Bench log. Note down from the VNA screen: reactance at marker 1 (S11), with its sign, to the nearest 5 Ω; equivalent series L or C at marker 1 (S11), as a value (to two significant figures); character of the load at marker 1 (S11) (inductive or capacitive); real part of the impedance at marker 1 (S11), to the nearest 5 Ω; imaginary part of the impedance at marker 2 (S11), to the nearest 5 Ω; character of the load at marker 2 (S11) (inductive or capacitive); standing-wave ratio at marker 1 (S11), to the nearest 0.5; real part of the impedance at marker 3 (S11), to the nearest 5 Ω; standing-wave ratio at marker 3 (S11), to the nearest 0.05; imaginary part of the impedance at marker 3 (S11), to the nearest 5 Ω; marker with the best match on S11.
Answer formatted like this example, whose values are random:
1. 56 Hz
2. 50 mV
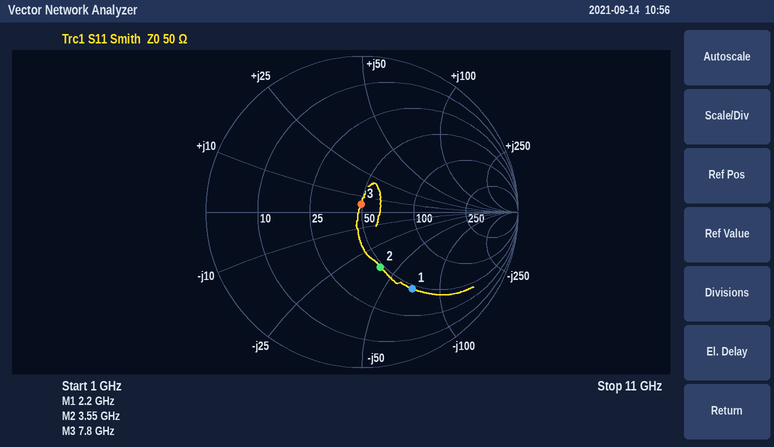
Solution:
1. -70 Ω
2. 1.0 pF
3. capacitive
4. 45 Ω
5. -40 Ω
6. capacitive
7. 4.0
8. 50 Ω
9. 1.10
10. +5 Ω
11. marker 3
